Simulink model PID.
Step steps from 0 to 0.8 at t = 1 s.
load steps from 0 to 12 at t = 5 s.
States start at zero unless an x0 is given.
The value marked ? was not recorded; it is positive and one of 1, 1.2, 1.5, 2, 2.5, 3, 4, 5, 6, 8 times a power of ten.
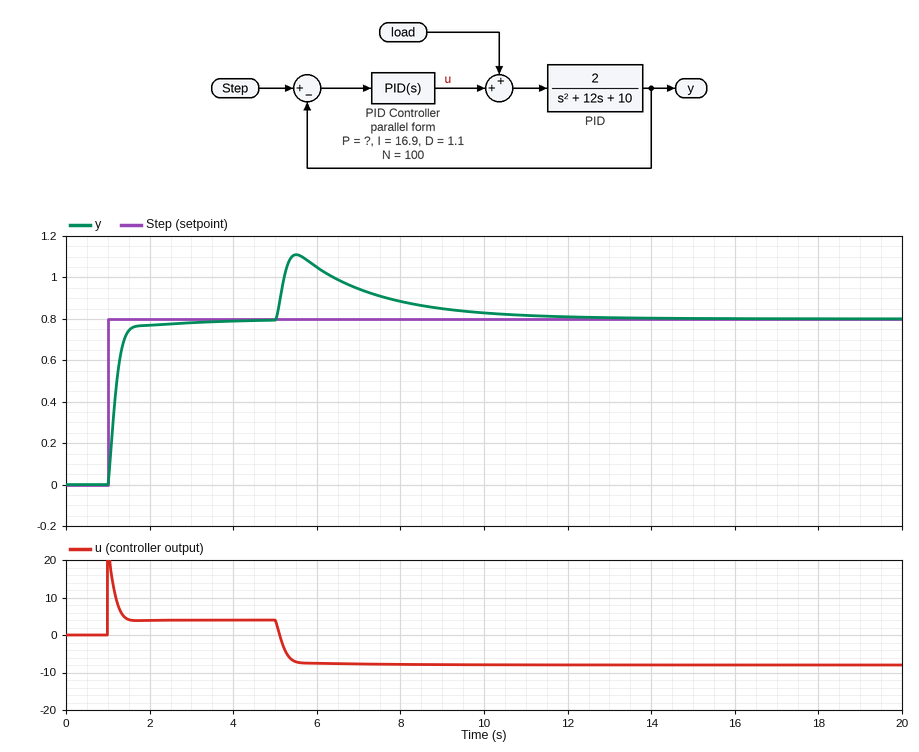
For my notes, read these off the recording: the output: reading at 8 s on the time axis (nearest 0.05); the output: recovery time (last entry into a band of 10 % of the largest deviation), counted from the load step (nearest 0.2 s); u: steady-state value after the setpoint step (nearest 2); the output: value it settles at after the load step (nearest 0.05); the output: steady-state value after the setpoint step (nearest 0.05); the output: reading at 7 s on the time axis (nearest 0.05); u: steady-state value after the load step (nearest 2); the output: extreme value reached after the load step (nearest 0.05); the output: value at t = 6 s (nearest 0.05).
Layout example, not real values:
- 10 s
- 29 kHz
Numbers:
- 0.90
- 4.8 s
- 4
- 0.80
- 0.80
- 0.95
- -8
- 1.10
- 1.05
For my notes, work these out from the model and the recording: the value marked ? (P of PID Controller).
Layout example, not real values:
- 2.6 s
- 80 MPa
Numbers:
- 30
